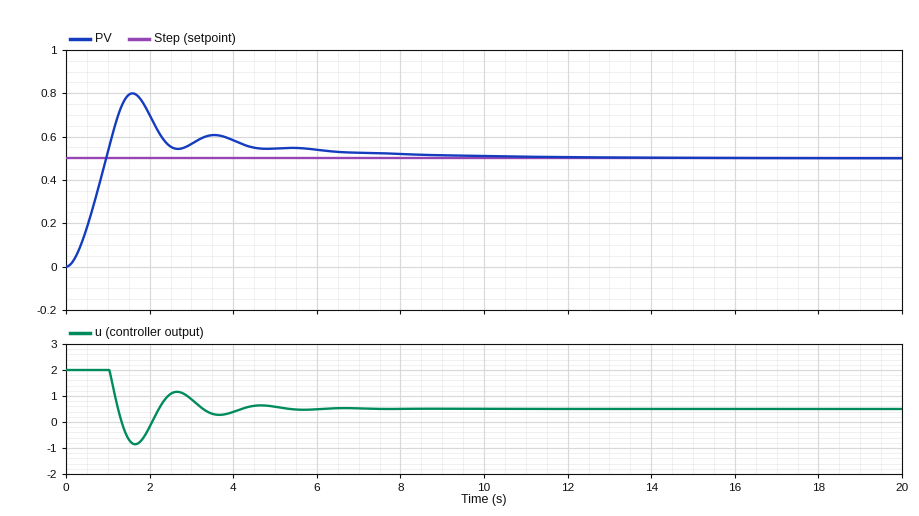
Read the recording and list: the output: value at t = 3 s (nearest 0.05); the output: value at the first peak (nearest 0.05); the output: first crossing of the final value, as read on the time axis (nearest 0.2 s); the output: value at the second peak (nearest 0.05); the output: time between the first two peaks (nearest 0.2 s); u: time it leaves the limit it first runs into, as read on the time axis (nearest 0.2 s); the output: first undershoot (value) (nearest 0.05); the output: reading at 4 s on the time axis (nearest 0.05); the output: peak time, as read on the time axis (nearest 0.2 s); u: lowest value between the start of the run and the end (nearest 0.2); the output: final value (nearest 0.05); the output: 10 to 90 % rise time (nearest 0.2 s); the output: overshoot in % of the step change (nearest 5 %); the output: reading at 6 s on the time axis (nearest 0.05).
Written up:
0.55
0.80
1.0 s
0.60
2.0 s
1.0 s
0.55
0.60
1.6 s
-0.8
0.50
0.6 s
60 %
0.55
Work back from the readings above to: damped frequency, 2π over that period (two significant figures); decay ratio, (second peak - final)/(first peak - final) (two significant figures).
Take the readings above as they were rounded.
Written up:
3.1 rad/s
0.33
